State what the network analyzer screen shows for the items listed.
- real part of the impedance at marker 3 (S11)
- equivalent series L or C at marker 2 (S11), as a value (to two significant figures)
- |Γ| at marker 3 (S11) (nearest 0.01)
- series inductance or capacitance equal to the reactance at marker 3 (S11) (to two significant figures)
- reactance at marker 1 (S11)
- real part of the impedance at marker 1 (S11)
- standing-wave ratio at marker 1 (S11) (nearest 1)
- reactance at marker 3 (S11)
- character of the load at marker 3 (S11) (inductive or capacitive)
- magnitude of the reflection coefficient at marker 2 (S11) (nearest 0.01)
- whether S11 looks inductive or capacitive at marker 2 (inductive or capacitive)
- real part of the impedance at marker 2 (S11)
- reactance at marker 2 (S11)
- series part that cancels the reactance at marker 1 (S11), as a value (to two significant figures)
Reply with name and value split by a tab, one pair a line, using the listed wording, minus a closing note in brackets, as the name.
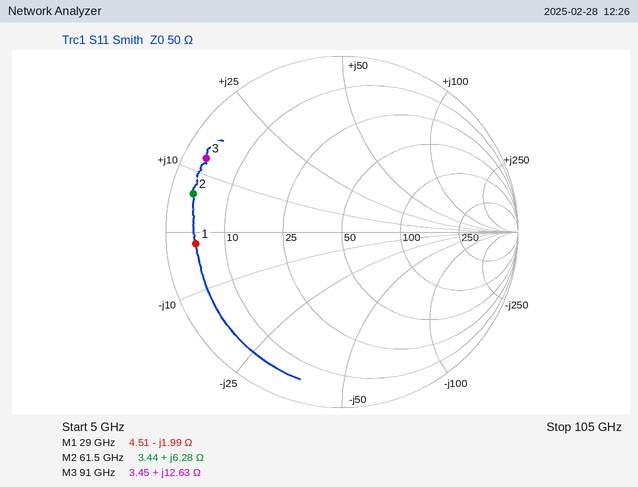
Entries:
real part of the impedance at marker 3	3.45 Ω
equivalent series L or C at marker 2 (S11), as a value	16 pH
|Γ| at marker 3 (S11)	0.88
series inductance or capacitance equal to the reactance at marker 3 (S11)	22 pH
reactance at marker 1	-1.99 Ω
real part of the impedance at marker 1	4.51 Ω
standing-wave ratio at marker 1 (S11)	11
reactance at marker 3	+12.63 Ω
character of the load at marker 3 (S11)	inductive
magnitude of the reflection coefficient at marker 2 (S11)	0.87
whether S11 looks inductive or capacitive at marker 2	inductive
real part of the impedance at marker 2	3.44 Ω
reactance at marker 2	+6.28 Ω
series part that cancels the reactance at marker 1 (S11), as a value	11 pH
